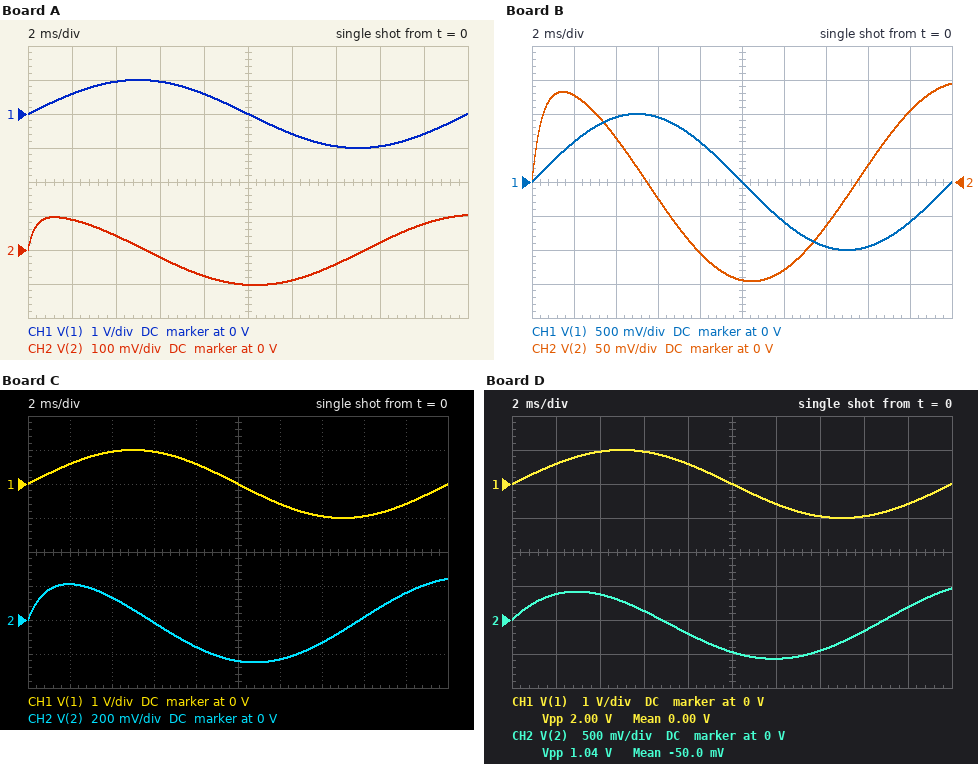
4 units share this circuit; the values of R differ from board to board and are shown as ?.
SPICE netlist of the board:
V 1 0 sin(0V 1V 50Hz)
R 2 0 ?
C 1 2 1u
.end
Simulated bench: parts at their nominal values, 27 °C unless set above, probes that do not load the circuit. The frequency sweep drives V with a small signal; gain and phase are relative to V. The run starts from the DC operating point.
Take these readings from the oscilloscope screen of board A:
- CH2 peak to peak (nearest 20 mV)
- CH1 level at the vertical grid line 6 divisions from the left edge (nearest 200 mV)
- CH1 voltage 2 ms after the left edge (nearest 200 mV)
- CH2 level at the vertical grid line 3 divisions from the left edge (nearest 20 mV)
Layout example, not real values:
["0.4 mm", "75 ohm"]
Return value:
["200 mV", "-600 mV", "600 mV", "-20 mV"]
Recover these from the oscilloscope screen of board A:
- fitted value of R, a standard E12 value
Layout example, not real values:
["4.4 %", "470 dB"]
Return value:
["330 Ω"]
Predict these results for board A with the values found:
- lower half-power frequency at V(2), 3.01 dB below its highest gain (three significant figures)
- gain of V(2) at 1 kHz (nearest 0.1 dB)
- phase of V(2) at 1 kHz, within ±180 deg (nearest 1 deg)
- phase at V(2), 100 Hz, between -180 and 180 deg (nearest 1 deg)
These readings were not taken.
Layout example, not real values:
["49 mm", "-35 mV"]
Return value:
["482 Hz", "-0.9 dB", "26 deg", "78 deg"]
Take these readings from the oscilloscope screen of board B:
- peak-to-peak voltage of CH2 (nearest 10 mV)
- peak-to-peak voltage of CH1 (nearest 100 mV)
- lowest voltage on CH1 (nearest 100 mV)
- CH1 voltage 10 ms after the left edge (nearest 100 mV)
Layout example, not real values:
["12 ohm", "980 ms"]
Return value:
["290 mV", "2.0 V", "-1.0 V", "0 V"]
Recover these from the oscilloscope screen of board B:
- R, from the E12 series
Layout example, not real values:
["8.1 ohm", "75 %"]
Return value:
["470 Ω"]
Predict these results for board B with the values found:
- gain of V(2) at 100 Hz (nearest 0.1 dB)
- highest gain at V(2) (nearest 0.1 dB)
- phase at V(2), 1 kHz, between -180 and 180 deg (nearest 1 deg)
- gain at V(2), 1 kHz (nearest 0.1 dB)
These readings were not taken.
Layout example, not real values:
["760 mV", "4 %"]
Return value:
["-11.0 dB", "0 dB", "19 deg", "-0.5 dB"]
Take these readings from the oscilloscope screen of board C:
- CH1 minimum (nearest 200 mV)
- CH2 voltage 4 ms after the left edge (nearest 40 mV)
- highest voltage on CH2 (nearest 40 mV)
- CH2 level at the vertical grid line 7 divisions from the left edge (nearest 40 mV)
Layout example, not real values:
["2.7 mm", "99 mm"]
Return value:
["-1.0 V", "120 mV", "240 mV", "-120 mV"]
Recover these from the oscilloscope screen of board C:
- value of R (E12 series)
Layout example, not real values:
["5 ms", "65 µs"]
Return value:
["820 Ω"]
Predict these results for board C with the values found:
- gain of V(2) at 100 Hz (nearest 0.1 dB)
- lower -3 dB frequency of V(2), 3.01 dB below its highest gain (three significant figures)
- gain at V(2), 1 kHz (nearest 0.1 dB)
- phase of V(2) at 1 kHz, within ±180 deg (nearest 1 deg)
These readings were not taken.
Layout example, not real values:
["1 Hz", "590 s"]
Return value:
["-6.8 dB", "194 Hz", "-0.2 dB", "11 deg"]
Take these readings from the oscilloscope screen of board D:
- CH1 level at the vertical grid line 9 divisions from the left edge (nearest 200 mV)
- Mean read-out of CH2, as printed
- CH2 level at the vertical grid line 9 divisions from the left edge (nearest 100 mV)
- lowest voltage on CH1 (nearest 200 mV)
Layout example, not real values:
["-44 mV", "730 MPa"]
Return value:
["-600 mV", "-50.0 mV", "200 mV", "-1.0 V"]
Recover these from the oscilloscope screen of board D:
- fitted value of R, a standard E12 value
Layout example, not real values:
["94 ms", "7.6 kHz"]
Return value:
["2.2 kΩ"]
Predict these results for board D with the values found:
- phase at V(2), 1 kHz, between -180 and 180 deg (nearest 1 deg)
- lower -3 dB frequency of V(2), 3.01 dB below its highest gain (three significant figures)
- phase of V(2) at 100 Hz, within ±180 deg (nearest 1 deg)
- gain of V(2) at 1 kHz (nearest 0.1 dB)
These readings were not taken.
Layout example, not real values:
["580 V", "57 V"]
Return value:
["4 deg", "72.3 Hz", "36 deg", "0 dB"]
